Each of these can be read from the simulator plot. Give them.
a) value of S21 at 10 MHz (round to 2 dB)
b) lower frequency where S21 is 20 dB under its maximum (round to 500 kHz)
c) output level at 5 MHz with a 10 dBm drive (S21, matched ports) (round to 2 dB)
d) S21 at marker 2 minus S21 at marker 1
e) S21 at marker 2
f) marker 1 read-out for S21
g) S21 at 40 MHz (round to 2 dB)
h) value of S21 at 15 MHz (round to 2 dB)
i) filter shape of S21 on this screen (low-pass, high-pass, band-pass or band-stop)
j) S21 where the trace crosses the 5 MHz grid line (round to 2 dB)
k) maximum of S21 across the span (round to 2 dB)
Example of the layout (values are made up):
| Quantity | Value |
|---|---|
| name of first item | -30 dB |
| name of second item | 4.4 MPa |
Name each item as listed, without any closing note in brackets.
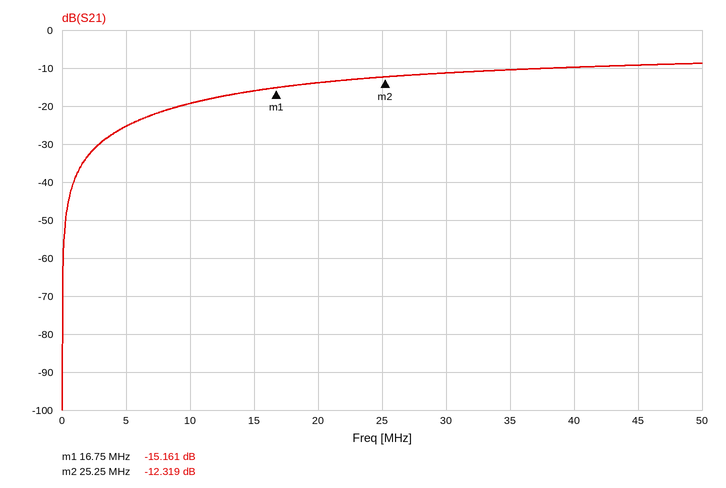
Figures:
| Quantity | Value |
|---|---|
| value of S21 at 10 MHz | -20 dB |
| lower frequency where S21 is 20 dB under its maximum | 3.5 MHz |
| output level at 5 MHz with a 10 dBm drive (S21, matched ports) | -16 dBm |
| S21 at marker 2 minus S21 at marker 1 | 2.842 dB |
| S21 at marker 2 | -12.319 dB |
| marker 1 read-out for S21 | -15.161 dB |
| S21 at 40 MHz | -10 dB |
| value of S21 at 15 MHz | -16 dB |
| filter shape of S21 on this screen | high-pass |
| S21 where the trace crosses the 5 MHz grid line | -26 dB |
| maximum of S21 across the span | -8 dB |
